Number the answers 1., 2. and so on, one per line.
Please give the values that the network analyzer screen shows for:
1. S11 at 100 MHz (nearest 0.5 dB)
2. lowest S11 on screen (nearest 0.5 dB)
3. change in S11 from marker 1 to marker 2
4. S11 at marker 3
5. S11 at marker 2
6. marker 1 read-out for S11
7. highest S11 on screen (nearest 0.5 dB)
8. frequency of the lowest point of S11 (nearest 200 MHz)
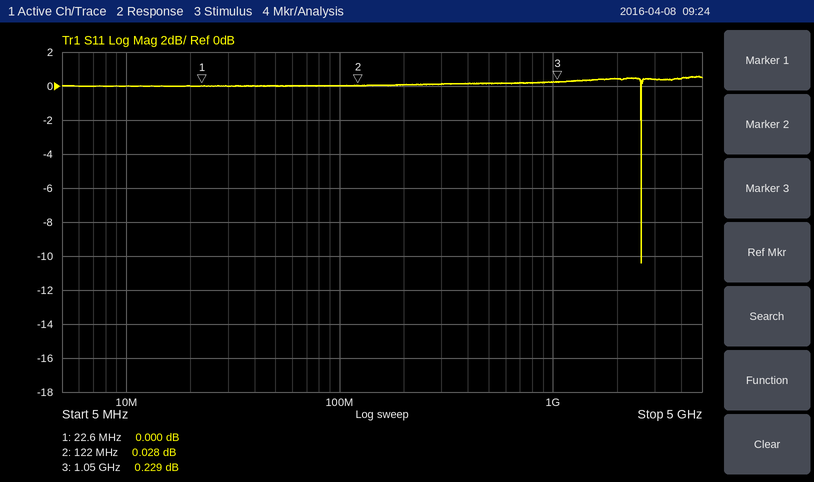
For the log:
1. 0.0 dB
2. -10.5 dB
3. 0.028 dB
4. 0.229 dB
5. 0.028 dB
6. 0.000 dB
7. 0.5 dB
8. 2.6 GHz
